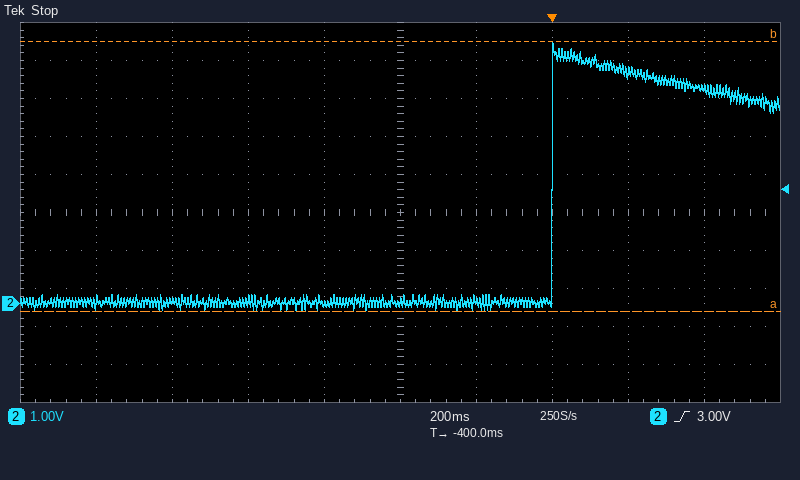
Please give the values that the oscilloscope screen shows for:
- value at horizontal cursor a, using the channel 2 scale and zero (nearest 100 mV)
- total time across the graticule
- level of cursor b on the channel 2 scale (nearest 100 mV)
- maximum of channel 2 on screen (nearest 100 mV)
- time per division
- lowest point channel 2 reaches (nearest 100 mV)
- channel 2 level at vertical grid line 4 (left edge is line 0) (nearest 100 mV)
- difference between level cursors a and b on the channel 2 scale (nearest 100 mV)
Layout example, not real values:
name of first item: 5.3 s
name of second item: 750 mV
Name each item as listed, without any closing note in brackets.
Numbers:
value at horizontal cursor a, using the channel 2 scale and zero: -200 mV
total time across the graticule: 2 s
level of cursor b on the channel 2 scale: 6.9 V
maximum of channel 2 on screen: 6.9 V
time per division: 200 ms
lowest point channel 2 reaches: -200 mV
channel 2 level at vertical grid line 4 (left edge is line 0): 0.0 V
difference between level cursors a and b on the channel 2 scale: 7.1 V
